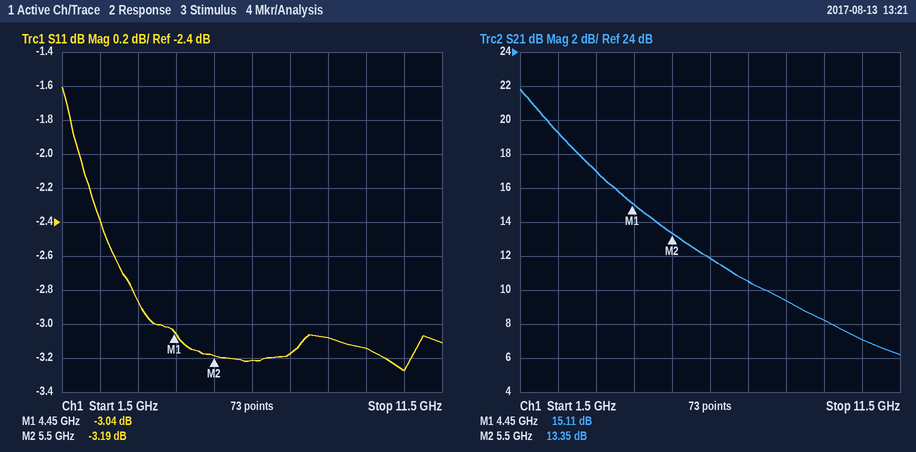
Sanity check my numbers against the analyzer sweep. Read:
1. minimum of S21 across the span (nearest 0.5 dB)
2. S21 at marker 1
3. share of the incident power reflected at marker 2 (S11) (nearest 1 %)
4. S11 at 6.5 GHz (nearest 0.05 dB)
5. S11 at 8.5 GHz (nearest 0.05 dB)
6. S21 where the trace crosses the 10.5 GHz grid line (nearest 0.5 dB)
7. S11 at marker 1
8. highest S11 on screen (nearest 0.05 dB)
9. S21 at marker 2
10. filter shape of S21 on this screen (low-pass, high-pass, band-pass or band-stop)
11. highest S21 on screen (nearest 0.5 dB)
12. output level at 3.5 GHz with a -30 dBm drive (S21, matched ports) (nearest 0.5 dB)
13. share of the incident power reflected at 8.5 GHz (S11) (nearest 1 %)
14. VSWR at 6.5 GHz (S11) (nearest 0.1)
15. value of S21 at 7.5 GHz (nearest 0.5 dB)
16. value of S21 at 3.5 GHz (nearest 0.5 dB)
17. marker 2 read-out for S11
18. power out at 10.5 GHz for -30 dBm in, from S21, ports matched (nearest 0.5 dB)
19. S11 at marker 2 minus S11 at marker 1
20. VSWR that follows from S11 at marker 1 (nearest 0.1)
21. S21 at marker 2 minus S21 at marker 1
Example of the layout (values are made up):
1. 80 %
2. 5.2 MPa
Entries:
1. 6.0 dB
2. 15.11 dB
3. 48 %
4. -3.20 dB
5. -3.10 dB
6. 7.0 dB
7. -3.04 dB
8. -1.60 dB
9. 13.35 dB
10. low-pass
11. 22.0 dB
12. -13.0 dBm
13. 49 %
14. 5.5
15. 10.5 dB
16. 17.0 dB
17. -3.19 dB
18. -23.0 dBm
19. -0.15 dB
20. 5.8
21. -1.76 dB
